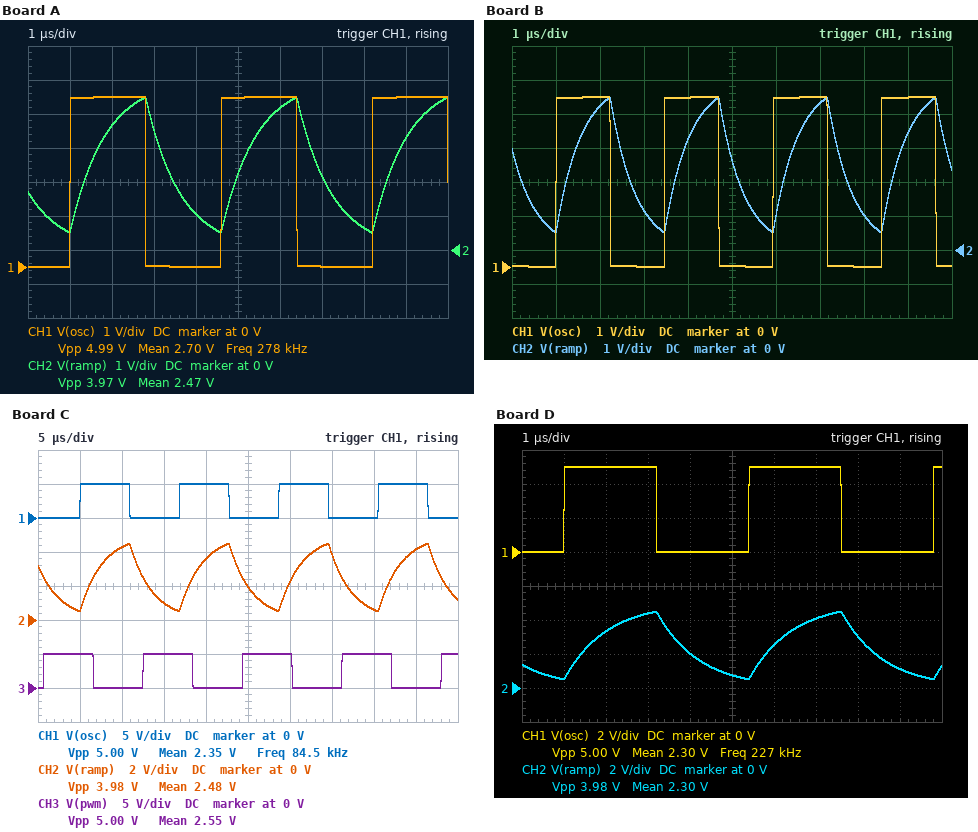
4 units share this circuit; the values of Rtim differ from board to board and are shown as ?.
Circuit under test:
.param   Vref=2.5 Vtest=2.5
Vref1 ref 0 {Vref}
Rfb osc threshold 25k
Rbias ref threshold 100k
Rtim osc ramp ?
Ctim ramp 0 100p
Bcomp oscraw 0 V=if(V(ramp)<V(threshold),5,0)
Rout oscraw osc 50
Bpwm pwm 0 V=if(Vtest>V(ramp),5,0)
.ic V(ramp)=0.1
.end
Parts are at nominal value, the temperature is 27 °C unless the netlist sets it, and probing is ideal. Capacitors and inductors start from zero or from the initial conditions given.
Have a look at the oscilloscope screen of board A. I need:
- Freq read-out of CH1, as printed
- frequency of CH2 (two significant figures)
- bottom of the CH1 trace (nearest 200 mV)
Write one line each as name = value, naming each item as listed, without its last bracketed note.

Freq read-out of CH1, as printed = 278 kHz
frequency of CH2 = 280 kHz
bottom of the CH1 trace = 0 V
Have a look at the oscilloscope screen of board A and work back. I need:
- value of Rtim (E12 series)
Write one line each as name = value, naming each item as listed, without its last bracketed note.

value of Rtim = 8.2 kΩ
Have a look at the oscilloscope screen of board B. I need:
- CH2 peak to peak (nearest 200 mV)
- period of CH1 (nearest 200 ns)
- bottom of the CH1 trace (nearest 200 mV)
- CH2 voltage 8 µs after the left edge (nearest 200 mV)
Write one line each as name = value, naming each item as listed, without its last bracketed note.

CH2 peak to peak = 4.0 V
period of CH1 = 2.4 µs
bottom of the CH1 trace = 0 V
CH2 voltage 8 µs after the left edge = 1.0 V
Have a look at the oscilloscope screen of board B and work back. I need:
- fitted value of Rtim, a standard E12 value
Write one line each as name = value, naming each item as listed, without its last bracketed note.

fitted value of Rtim, a standard E12 value = 5.6 kΩ
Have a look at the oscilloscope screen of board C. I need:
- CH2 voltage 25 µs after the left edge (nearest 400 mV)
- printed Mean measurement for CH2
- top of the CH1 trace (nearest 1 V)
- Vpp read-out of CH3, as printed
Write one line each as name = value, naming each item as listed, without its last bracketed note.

CH2 voltage 25 µs after the left edge = 2.0 V
printed Mean measurement for CH2 = 2.48 V
top of the CH1 trace = 5 V
Vpp read-out of CH3, as printed = 5.00 V
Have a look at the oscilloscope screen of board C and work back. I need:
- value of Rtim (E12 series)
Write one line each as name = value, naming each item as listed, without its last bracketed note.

value of Rtim = 27 kΩ
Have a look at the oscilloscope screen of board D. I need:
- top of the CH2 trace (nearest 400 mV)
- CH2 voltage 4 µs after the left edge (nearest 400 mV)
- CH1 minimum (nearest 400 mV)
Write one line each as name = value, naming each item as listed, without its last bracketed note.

top of the CH2 trace = 4.4 V
CH2 voltage 4 µs after the left edge = 2.0 V
CH1 minimum = 0 V
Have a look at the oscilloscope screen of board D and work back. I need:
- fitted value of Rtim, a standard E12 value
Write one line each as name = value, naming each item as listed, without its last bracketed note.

fitted value of Rtim, a standard E12 value = 10 kΩ
